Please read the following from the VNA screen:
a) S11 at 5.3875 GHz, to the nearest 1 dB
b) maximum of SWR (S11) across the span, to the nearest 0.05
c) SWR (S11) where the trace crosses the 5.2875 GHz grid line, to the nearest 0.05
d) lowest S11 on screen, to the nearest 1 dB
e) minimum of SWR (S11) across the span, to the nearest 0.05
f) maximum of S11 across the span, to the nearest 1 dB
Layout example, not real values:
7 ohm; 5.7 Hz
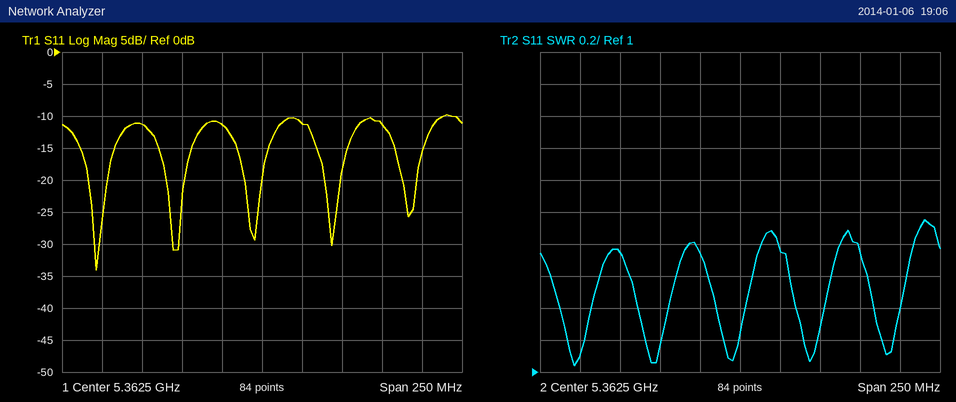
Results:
-11 dB; 1.95; 1.75; -34 dB; 1.05; -10 dB
